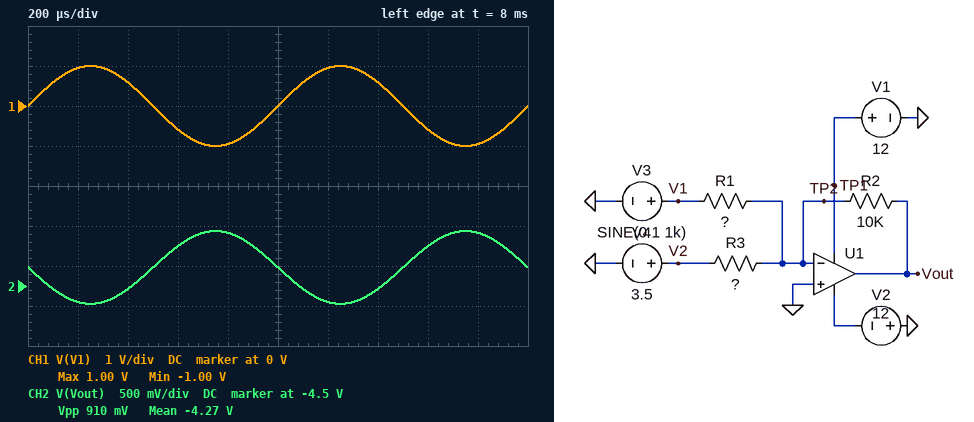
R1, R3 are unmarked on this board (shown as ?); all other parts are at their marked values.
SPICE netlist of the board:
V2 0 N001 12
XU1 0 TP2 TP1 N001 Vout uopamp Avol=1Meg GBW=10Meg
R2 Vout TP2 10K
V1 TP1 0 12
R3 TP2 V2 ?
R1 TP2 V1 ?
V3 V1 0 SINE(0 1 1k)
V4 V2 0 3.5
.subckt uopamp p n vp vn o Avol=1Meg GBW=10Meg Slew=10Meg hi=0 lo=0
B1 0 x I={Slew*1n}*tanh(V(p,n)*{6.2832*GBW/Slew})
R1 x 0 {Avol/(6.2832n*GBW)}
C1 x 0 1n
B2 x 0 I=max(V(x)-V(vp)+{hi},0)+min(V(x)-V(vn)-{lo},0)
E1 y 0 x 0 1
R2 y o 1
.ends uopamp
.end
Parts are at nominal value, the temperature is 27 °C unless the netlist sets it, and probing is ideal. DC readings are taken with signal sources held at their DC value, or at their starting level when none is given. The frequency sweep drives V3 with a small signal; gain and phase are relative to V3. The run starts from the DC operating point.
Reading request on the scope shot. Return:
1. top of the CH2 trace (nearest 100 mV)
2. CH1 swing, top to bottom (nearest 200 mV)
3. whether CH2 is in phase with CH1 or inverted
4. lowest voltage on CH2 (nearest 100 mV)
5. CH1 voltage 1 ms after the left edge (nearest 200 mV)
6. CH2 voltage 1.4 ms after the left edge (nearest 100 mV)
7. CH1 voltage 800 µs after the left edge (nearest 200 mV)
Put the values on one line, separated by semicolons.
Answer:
-3.8 V; 2.0 V; inverted; -4.7 V; 0 V; -4.5 V; -1.0 V
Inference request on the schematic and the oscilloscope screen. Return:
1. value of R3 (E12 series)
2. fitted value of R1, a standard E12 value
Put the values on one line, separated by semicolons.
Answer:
8.2 kΩ; 22 kΩ
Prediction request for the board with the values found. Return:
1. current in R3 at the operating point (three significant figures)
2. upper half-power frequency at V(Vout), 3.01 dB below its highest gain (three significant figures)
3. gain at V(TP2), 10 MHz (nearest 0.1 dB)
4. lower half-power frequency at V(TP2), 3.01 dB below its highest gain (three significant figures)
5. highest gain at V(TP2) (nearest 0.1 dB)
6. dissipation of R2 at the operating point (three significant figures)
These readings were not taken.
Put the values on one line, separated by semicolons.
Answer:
427 µA; 3.74 MHz; -16.0 dB; 3.74 MHz; -15.4 dB; 1.82 mW
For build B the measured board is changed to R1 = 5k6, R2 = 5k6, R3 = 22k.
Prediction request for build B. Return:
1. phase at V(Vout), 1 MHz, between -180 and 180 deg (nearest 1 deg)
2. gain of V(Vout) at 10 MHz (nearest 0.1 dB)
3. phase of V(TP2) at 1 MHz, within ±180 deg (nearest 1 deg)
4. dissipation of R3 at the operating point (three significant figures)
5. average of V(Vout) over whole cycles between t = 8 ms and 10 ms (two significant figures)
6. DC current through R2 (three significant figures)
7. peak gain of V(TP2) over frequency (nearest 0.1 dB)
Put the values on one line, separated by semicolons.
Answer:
167 deg; -7.8 dB; 77 deg; 557 µW; -890 mV; 159 µA; -7.1 dB
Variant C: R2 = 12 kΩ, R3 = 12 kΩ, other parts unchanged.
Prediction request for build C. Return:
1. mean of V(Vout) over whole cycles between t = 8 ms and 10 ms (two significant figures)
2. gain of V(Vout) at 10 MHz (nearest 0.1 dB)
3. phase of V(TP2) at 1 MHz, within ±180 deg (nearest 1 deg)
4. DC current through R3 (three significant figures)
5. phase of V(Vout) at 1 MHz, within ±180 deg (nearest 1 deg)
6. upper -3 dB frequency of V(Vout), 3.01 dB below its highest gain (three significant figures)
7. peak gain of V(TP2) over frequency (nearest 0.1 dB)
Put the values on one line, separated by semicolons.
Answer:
-3.5 V; -14.0 dB; 76 deg; 292 µA; 166 deg; 3.93 MHz; -13.4 dB
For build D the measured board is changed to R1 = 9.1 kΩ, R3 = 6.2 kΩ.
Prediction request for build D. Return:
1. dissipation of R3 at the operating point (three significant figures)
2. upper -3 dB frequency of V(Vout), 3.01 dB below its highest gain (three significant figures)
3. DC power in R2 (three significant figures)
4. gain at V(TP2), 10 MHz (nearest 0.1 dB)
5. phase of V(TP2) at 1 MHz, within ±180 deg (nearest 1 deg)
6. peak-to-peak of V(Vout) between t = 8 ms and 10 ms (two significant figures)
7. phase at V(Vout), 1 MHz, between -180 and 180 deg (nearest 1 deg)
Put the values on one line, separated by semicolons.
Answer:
1.98 mW; 2.69 MHz; 3.19 mW; -10.9 dB; 70 deg; 2.2 V; 160 deg
